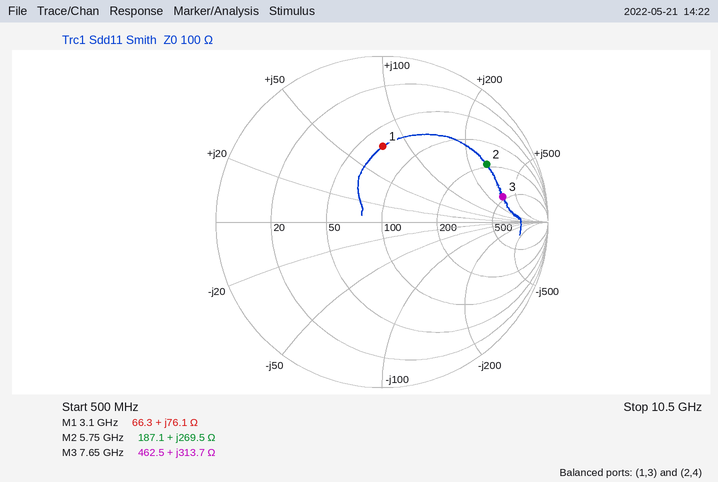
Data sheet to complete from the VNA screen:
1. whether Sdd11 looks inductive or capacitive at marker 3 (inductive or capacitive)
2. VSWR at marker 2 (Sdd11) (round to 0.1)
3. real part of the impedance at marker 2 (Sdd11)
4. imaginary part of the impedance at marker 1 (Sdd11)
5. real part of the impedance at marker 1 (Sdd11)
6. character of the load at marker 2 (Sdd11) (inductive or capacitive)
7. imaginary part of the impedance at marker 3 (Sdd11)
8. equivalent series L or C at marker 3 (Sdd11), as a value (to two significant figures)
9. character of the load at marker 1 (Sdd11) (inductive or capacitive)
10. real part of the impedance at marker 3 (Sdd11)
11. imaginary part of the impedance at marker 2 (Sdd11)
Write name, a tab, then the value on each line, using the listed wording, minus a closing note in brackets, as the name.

whether Sdd11 looks inductive or capacitive at marker 3	inductive
VSWR at marker 2 (Sdd11)	6.1
real part of the impedance at marker 2	187.1 Ω
imaginary part of the impedance at marker 1	+76.1 Ω
real part of the impedance at marker 1	66.3 Ω
character of the load at marker 2 (Sdd11)	inductive
imaginary part of the impedance at marker 3	+313.7 Ω
equivalent series L or C at marker 3 (Sdd11), as a value	6.5 nH
character of the load at marker 1 (Sdd11)	inductive
real part of the impedance at marker 3	462.5 Ω
imaginary part of the impedance at marker 2	+269.5 Ω
